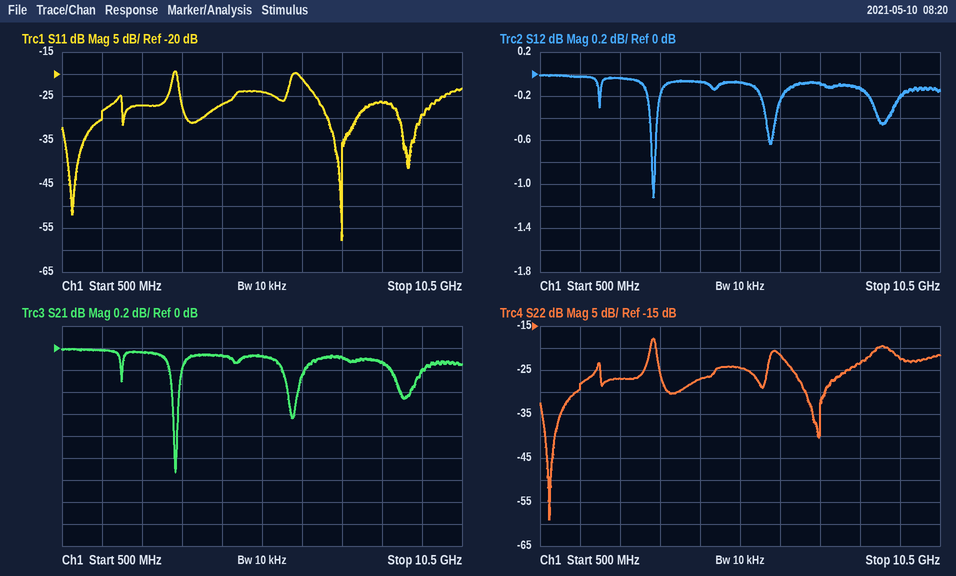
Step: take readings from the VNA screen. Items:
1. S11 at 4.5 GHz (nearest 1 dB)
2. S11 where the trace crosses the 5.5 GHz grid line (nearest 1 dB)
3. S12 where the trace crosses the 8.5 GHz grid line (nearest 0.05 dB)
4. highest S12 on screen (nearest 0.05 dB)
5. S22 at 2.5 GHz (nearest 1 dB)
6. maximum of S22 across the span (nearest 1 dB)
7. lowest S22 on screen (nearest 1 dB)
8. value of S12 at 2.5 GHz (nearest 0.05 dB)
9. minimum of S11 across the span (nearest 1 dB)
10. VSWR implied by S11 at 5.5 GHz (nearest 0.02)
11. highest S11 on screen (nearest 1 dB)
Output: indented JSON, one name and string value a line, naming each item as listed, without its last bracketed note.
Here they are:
{
  "S11 at 4.5 GHz": "-27 dB",
  "S11 where the trace crosses the 5.5 GHz grid line": "-24 dB",
  "S12 where the trace crosses the 8.5 GHz grid line": "-0.15 dB",
  "highest S12 on screen": "0.00 dB",
  "S22 at 2.5 GHz": "-27 dB",
  "maximum of S22 across the span": "-18 dB",
  "lowest S22 on screen": "-59 dB",
  "value of S12 at 2.5 GHz": "-0.05 dB",
  "minimum of S11 across the span": "-58 dB",
  "VSWR implied by S11 at 5.5 GHz": "1.14",
  "highest S11 on screen": "-19 dB"
}
